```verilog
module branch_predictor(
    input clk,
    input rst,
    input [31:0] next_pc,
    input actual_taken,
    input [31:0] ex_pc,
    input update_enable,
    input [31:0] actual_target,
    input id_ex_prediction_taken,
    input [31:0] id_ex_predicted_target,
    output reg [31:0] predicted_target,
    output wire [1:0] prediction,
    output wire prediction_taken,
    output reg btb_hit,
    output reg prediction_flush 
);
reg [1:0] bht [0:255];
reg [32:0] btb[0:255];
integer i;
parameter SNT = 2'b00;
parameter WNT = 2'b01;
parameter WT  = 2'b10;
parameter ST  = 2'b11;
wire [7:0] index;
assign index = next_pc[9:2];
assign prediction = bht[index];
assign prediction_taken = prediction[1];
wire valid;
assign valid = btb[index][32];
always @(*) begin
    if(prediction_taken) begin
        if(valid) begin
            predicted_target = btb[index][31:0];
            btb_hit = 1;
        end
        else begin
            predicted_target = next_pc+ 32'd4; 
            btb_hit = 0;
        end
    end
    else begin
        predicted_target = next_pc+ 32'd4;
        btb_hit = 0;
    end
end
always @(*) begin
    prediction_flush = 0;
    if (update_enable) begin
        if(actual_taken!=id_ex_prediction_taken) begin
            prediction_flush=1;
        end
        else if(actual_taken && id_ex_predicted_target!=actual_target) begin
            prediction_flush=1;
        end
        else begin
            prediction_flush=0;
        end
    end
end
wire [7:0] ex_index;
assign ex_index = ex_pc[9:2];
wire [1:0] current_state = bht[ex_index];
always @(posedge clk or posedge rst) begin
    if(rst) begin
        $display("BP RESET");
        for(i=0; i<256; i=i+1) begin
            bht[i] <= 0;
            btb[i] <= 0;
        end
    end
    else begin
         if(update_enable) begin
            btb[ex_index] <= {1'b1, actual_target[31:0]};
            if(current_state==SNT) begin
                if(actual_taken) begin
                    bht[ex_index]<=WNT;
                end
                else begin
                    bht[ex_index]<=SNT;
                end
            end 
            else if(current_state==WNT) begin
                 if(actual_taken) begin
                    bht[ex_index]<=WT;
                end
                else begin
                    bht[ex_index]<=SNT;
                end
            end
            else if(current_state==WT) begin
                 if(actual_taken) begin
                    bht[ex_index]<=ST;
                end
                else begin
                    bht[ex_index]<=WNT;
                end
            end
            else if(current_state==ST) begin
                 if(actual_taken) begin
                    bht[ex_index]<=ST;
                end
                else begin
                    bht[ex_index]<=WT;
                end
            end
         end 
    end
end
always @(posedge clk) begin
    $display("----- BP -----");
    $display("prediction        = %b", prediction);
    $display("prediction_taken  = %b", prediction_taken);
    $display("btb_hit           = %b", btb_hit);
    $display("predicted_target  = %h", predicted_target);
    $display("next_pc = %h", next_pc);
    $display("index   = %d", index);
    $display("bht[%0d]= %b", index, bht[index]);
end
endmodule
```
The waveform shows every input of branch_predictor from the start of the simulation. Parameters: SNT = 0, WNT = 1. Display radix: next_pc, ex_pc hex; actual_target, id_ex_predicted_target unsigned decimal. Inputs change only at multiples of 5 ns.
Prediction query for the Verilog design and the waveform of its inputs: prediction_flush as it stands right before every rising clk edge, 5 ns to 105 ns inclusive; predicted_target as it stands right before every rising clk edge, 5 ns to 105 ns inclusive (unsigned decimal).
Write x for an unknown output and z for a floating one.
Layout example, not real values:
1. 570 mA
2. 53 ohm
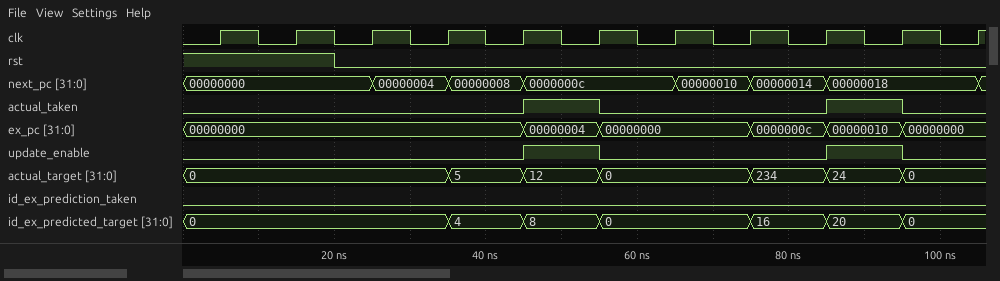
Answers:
1. 0 0 0 0 0 1 0 0 0 1 0
2. 4, 4, 4, 8, 12, 16, 16, 20, 24, 28, 28
